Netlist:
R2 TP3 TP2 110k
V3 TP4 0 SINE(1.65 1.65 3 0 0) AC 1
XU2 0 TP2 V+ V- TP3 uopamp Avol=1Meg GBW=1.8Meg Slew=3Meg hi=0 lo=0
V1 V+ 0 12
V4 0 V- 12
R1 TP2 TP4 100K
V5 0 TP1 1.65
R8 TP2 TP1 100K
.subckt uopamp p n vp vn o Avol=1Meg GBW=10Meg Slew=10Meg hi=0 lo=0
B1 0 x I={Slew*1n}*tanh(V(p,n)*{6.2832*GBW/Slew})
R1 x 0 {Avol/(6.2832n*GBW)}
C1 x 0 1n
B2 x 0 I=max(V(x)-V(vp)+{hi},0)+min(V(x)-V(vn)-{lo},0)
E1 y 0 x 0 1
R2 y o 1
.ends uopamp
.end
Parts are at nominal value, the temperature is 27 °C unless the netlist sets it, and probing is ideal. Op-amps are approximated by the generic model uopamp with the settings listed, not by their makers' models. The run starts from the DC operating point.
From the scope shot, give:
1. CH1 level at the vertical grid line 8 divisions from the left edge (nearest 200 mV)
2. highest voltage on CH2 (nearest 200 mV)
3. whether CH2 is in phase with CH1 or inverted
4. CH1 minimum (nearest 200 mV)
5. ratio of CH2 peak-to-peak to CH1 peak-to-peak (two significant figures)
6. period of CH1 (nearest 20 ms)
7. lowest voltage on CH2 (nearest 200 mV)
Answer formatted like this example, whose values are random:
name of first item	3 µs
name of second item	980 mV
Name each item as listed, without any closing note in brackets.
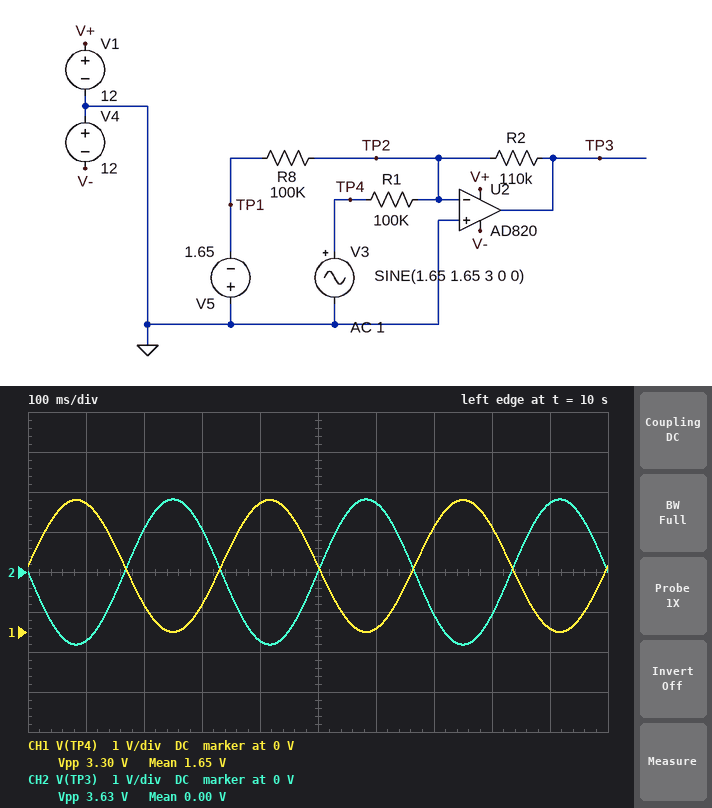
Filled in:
CH1 level at the vertical grid line 8 divisions from the left edge	2.6 V
highest voltage on CH2	1.8 V
whether CH2 is in phase with CH1 or inverted	inverted
CH1 minimum	0 V
ratio of CH2 peak-to-peak to CH1 peak-to-peak	1.1
period of CH1	340 ms
lowest voltage on CH2	-1.8 V
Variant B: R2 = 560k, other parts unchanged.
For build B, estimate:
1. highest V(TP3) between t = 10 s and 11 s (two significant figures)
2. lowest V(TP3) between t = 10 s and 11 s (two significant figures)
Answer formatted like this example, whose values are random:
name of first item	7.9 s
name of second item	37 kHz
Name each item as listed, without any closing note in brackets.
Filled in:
highest V(TP3) between t = 10 s and 11 s	9.2 V
lowest V(TP3) between t = 10 s and 11 s	-9.2 V
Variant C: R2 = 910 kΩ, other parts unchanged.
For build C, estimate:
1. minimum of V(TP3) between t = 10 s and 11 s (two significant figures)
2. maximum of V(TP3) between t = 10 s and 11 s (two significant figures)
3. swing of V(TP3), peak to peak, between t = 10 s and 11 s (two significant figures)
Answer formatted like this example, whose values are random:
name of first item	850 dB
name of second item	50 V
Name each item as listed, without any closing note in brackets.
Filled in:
minimum of V(TP3) between t = 10 s and 11 s	-12 V
maximum of V(TP3) between t = 10 s and 11 s	12 V
swing of V(TP3), peak to peak, between t = 10 s and 11 s	24 V
